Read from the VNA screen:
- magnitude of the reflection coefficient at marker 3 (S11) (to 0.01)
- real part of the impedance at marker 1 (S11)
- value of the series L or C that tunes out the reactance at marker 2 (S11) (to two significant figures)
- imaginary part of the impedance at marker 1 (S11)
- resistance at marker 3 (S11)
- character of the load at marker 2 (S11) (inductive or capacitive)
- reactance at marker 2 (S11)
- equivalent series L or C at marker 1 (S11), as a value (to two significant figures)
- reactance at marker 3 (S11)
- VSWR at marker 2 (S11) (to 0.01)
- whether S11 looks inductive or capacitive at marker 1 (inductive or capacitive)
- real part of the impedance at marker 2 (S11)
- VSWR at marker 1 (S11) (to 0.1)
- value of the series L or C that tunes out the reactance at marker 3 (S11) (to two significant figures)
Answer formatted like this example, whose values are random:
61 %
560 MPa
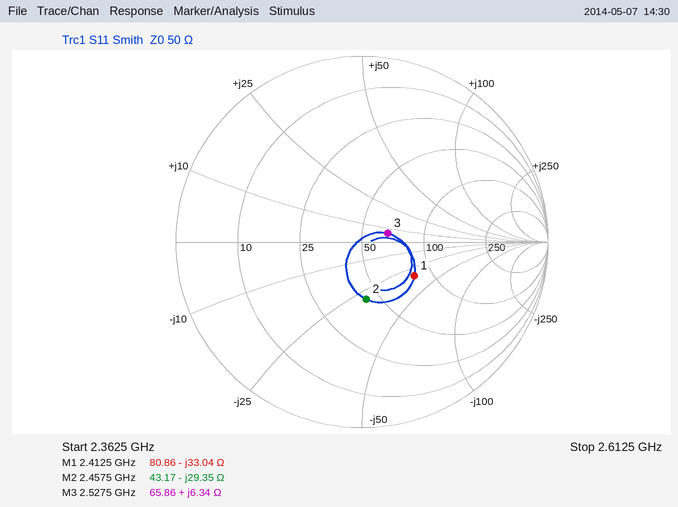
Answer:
0.15
80.86 Ω
1.9 nH
-33.04 Ω
65.86 Ω
capacitive
-29.35 Ω
2.0 pF
+6.34 Ω
1.89
capacitive
43.17 Ω
2.0
9.9 pF
